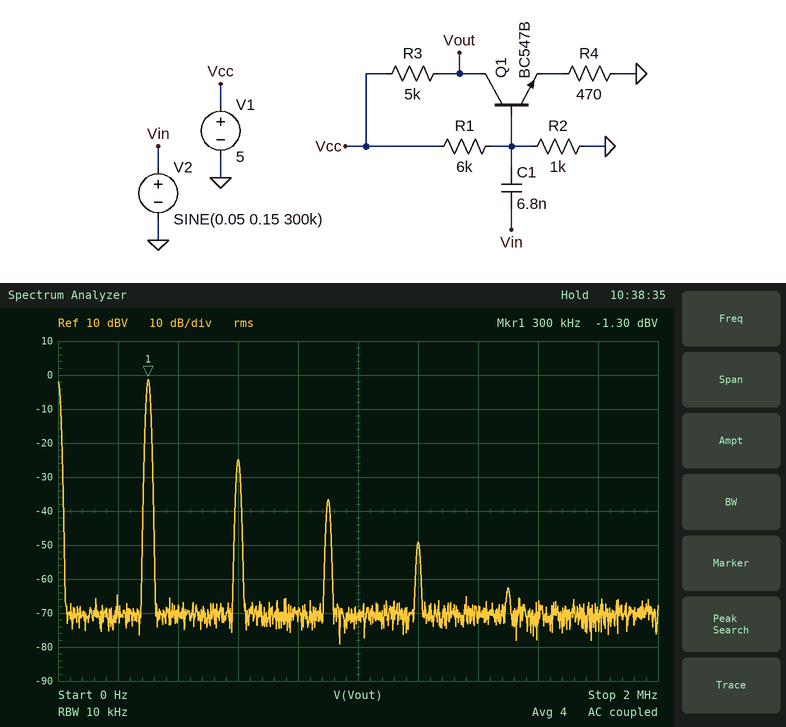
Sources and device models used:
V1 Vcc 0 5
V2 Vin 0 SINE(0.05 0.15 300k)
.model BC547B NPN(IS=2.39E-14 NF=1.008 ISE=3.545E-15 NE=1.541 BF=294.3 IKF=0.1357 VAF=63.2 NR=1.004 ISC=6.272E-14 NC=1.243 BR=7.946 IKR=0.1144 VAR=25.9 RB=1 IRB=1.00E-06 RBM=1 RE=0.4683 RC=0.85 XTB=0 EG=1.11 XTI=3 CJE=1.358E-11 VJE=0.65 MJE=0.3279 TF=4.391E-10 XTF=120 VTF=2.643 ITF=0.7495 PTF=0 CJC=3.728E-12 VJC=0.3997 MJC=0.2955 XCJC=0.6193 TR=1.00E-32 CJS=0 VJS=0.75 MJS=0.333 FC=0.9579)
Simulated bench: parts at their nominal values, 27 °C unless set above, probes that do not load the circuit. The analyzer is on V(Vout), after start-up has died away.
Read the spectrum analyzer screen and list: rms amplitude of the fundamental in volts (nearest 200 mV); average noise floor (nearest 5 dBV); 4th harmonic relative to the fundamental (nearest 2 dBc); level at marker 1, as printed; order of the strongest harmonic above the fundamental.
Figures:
800 mV
-70 dBV
-48 dBc
-1.30 dBV
2
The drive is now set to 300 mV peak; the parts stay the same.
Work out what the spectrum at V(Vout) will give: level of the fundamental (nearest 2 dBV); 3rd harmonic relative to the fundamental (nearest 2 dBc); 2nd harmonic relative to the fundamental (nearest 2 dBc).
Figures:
4 dBV
-24 dBc
-14 dBc
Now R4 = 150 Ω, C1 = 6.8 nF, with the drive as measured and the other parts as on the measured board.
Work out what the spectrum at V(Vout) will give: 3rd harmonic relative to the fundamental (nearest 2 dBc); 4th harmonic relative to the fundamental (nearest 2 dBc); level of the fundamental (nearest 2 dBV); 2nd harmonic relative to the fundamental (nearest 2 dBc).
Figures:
-18 dBc
-28 dBc
6 dBV
-34 dBc
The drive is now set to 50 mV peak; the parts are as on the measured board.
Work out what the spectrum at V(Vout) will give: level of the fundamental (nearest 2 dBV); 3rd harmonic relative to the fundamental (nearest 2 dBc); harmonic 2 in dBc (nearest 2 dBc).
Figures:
-10 dBV
-56 dBc
-36 dBc
